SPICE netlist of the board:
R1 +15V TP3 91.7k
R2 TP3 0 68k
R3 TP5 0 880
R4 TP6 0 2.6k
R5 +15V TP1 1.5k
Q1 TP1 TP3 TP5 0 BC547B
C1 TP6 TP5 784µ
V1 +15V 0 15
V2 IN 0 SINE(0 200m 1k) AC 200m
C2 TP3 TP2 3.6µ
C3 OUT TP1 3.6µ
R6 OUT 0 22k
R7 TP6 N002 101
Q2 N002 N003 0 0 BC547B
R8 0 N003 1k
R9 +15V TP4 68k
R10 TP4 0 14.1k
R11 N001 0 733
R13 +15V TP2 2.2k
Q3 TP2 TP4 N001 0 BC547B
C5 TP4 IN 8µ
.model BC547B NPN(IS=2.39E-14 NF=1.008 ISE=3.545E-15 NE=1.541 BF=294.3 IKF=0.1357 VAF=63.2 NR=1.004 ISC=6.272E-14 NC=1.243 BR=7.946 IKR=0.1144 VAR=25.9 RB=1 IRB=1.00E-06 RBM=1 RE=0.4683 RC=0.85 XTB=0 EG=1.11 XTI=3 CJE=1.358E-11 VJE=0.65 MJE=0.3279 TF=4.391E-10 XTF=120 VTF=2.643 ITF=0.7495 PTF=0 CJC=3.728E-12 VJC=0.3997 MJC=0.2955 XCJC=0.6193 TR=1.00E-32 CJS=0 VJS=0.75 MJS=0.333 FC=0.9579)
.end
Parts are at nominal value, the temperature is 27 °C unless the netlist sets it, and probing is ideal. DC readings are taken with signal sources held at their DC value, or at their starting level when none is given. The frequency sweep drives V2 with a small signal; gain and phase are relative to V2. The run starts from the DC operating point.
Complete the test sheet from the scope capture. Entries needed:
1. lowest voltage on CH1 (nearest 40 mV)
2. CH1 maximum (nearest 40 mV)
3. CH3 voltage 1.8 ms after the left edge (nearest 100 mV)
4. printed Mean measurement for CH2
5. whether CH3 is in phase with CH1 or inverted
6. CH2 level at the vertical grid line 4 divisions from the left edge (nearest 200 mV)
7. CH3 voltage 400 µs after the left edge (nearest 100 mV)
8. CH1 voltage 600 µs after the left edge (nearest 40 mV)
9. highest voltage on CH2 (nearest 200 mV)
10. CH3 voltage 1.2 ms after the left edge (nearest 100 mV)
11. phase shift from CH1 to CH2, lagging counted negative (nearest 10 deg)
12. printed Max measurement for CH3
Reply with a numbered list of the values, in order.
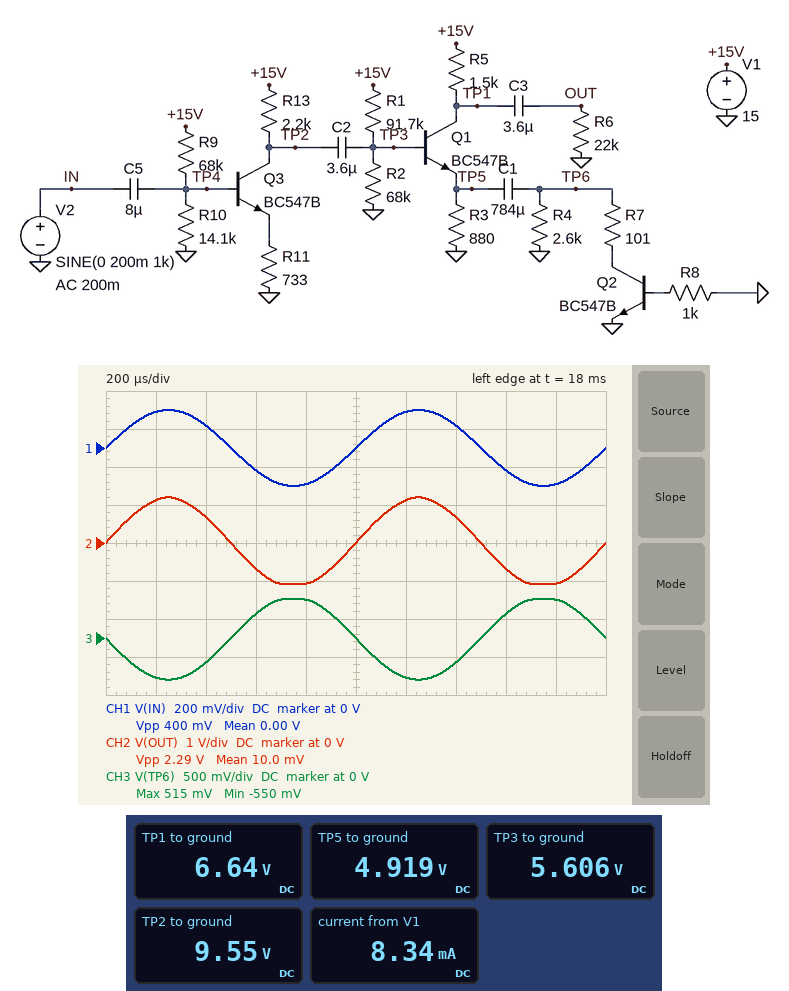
1. -200 mV
2. 200 mV
3. 500 mV
4. 10.0 mV
5. inverted
6. -1.0 V
7. -300 mV
8. -120 mV
9. 1.2 V
10. -500 mV
11. 0 deg
12. 515 mV
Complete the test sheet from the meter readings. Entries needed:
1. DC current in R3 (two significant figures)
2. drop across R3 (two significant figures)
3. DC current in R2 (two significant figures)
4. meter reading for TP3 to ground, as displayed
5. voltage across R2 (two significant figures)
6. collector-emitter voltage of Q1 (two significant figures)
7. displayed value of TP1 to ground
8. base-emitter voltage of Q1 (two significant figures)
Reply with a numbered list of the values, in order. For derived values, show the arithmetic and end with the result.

1. (4.919 V) / 880 Ω = 5.6 mA
2. 4.919 V = 4.9 V
3. (5.606 V) / 68 kΩ = 82 µA
4. 5.606 V
5. 5.606 V = 5.6 V
6. 6.64 V - 4.919 V = 1.7 V
7. 6.64 V
8. 5.606 V - 4.919 V = 690 mV
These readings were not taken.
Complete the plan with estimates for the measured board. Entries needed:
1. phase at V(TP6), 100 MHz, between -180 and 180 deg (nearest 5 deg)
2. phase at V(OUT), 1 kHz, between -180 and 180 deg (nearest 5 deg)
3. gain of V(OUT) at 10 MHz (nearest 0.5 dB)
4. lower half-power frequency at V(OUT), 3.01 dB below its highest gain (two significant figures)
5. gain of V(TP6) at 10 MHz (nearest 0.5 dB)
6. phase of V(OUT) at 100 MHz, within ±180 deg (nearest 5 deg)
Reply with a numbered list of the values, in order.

1. 65 deg
2. 0 deg
3. 10.0 dB
4. 3.3 Hz
5. 3.5 dB
6. 155 deg
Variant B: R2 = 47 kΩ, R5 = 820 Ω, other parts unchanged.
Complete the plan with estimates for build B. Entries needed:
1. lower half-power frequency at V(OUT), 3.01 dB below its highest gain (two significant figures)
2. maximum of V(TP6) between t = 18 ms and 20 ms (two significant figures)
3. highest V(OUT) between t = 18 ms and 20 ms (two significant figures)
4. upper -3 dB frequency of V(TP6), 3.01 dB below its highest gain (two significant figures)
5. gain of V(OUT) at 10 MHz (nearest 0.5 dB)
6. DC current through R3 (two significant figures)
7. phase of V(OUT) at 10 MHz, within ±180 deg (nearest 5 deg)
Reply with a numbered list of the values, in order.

1. 3.5 Hz
2. 540 mV
3. 660 mV
4. 12 MHz
5. 8.0 dB
6. 4.5 mA
7. -50 deg
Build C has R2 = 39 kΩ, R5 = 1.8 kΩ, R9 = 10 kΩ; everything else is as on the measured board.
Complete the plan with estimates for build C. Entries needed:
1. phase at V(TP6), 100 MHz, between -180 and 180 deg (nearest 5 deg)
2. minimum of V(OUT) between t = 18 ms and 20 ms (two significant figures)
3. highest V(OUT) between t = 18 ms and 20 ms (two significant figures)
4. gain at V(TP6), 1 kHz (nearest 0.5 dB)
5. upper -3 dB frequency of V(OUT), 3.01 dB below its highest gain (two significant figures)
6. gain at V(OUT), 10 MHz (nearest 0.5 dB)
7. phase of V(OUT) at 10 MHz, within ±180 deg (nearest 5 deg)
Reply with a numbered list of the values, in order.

1. 0 deg
2. -460 mV
3. 450 mV
4. -1.0 dB
5. 97 MHz
6. 7.5 dB
7. 170 deg
